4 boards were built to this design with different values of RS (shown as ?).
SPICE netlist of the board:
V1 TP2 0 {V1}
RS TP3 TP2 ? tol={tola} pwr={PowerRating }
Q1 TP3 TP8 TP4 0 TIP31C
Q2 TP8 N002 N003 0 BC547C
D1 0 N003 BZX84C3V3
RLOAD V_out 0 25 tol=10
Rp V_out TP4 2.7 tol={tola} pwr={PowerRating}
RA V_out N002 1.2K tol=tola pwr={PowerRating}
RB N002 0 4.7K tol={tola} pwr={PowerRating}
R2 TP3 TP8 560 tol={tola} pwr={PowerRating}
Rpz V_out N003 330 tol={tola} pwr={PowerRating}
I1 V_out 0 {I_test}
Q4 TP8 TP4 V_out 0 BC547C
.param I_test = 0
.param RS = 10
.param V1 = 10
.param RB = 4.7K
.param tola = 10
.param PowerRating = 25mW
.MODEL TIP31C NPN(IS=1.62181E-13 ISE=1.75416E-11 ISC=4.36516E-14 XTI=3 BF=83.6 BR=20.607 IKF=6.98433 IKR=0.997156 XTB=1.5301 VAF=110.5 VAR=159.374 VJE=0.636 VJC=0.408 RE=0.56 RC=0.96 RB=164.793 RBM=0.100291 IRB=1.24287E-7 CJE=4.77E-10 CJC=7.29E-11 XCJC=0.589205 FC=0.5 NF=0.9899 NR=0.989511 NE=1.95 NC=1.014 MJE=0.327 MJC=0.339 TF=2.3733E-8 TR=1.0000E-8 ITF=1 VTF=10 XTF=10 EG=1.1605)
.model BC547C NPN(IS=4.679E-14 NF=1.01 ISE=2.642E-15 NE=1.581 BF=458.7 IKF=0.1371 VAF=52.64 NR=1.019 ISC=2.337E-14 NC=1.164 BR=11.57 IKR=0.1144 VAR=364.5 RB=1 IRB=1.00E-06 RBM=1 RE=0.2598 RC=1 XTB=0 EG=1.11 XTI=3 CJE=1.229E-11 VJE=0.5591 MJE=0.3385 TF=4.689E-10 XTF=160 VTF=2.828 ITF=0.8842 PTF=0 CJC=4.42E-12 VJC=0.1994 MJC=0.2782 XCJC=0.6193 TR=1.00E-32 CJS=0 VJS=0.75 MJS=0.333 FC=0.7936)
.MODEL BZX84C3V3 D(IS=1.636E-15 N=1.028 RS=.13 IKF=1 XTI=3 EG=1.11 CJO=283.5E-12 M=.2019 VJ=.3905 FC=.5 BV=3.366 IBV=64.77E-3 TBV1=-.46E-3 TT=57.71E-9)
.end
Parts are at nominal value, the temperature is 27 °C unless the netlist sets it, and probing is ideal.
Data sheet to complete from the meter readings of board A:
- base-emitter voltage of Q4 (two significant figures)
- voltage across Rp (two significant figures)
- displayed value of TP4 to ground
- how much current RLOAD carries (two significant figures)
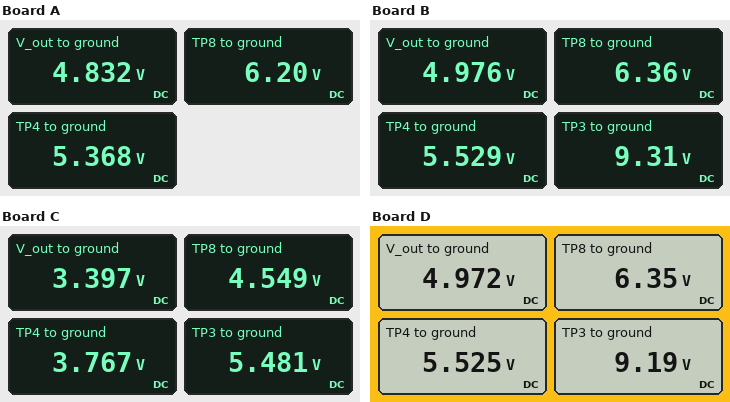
540 mV
540 mV
5.368 V
190 mA
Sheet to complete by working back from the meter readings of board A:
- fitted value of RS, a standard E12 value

12 Ω
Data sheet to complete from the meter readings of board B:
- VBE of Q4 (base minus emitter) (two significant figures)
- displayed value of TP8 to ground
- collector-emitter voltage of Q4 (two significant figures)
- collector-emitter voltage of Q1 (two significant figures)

550 mV
6.36 V
1.4 V
3.8 V
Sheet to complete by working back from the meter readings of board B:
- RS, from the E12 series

3.3 Ω
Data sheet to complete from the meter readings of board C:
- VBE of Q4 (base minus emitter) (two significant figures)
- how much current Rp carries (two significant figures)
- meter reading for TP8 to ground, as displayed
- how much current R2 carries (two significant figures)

370 mV
140 mA
4.549 V
1.7 mA
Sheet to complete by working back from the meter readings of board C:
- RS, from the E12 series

33 Ω
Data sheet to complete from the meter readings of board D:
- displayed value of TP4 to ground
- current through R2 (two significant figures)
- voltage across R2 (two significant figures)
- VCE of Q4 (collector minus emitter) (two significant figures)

5.525 V
5.1 mA
2.8 V
1.4 V
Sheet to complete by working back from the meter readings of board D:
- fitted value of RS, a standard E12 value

3.9 Ω
